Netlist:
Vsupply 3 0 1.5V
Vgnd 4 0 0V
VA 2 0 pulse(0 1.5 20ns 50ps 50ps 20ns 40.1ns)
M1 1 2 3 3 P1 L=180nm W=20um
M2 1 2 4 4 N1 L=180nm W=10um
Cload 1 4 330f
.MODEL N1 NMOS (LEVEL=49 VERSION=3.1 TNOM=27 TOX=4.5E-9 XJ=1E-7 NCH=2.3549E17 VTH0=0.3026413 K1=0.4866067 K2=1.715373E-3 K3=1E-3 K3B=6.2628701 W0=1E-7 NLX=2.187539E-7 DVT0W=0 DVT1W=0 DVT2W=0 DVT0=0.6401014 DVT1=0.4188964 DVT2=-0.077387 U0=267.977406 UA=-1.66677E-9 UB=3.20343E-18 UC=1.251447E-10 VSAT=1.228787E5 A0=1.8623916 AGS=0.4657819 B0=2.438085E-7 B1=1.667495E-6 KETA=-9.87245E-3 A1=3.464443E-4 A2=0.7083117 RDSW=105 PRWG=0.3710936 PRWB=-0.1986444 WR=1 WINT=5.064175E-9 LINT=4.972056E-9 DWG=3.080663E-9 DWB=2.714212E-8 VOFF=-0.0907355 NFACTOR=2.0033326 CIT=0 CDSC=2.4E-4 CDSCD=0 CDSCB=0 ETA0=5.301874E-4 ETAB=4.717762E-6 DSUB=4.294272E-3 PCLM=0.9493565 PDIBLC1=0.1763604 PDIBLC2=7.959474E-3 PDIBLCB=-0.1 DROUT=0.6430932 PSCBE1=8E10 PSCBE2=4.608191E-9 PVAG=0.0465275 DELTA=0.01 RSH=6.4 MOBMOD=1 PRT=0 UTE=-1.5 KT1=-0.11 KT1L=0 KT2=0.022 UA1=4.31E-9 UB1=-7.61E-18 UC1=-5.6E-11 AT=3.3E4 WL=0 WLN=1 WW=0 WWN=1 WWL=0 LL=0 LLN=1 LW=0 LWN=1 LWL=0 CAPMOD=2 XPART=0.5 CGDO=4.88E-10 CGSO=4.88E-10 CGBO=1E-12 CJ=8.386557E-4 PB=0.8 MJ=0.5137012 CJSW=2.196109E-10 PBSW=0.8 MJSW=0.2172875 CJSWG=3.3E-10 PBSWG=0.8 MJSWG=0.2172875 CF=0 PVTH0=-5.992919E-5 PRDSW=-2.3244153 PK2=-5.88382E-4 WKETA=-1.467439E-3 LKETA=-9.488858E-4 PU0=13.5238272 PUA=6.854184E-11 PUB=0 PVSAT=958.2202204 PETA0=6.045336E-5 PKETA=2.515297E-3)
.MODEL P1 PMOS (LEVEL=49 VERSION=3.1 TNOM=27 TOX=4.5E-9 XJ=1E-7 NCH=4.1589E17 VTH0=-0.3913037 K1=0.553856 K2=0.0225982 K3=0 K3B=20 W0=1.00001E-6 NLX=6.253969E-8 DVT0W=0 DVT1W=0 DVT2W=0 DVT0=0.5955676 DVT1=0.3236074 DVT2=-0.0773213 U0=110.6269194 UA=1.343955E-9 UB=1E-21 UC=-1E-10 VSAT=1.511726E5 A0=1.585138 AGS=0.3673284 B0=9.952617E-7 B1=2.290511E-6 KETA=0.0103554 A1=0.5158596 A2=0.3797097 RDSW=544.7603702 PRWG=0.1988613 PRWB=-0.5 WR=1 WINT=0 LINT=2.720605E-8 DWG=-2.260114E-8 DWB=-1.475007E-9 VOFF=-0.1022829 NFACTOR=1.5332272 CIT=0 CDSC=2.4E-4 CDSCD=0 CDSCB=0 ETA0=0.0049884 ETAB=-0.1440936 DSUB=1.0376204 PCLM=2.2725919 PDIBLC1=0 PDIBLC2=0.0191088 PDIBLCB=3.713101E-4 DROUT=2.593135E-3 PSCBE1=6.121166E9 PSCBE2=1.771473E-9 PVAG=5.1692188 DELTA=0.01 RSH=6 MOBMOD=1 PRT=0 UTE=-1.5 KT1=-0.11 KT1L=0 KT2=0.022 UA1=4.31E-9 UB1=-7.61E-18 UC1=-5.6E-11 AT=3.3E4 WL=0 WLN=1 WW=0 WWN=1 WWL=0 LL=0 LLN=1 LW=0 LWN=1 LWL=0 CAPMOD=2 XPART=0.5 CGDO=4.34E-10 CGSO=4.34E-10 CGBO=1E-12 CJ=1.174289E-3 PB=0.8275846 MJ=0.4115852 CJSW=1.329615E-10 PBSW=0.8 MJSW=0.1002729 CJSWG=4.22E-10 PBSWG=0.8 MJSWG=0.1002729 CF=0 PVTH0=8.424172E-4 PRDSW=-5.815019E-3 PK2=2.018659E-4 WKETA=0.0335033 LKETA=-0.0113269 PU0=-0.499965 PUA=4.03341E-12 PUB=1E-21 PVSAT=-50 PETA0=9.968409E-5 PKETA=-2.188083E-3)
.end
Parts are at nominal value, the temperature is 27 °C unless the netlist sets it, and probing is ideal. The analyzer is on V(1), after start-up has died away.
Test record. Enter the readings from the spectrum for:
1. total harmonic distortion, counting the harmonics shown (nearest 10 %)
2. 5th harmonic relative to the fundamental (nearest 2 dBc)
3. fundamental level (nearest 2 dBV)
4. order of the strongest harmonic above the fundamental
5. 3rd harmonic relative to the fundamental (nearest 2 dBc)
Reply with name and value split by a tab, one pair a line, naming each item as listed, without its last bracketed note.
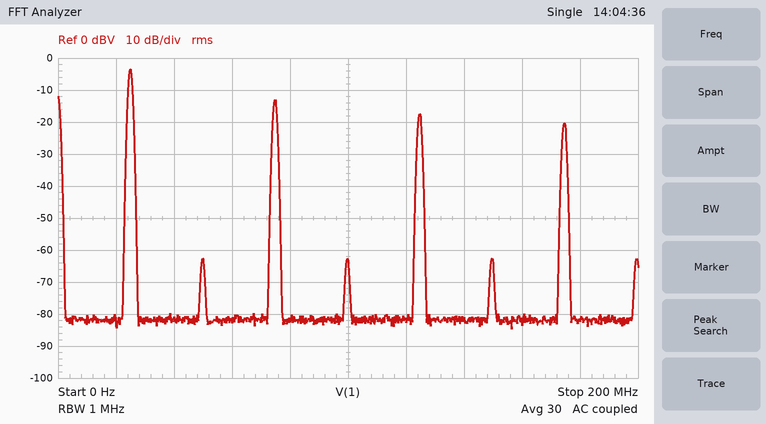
total harmonic distortion, counting the harmonics shown	40 %
5th harmonic relative to the fundamental	-14 dBc
fundamental level	-4 dBV
order of the strongest harmonic above the fundamental	3
3rd harmonic relative to the fundamental	-10 dBc
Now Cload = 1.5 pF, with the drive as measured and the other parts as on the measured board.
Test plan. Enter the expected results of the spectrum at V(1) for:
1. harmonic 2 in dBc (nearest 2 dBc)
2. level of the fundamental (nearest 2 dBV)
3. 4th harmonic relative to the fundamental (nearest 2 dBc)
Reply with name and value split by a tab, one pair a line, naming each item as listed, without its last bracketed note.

harmonic 2 in dBc	-48 dBc
level of the fundamental	-4 dBV
4th harmonic relative to the fundamental	-48 dBc
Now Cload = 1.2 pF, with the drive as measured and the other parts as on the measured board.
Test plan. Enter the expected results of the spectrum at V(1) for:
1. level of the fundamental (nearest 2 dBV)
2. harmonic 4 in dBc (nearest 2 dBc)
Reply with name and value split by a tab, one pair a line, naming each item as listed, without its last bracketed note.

level of the fundamental	-4 dBV
harmonic 4 in dBc	-50 dBc
